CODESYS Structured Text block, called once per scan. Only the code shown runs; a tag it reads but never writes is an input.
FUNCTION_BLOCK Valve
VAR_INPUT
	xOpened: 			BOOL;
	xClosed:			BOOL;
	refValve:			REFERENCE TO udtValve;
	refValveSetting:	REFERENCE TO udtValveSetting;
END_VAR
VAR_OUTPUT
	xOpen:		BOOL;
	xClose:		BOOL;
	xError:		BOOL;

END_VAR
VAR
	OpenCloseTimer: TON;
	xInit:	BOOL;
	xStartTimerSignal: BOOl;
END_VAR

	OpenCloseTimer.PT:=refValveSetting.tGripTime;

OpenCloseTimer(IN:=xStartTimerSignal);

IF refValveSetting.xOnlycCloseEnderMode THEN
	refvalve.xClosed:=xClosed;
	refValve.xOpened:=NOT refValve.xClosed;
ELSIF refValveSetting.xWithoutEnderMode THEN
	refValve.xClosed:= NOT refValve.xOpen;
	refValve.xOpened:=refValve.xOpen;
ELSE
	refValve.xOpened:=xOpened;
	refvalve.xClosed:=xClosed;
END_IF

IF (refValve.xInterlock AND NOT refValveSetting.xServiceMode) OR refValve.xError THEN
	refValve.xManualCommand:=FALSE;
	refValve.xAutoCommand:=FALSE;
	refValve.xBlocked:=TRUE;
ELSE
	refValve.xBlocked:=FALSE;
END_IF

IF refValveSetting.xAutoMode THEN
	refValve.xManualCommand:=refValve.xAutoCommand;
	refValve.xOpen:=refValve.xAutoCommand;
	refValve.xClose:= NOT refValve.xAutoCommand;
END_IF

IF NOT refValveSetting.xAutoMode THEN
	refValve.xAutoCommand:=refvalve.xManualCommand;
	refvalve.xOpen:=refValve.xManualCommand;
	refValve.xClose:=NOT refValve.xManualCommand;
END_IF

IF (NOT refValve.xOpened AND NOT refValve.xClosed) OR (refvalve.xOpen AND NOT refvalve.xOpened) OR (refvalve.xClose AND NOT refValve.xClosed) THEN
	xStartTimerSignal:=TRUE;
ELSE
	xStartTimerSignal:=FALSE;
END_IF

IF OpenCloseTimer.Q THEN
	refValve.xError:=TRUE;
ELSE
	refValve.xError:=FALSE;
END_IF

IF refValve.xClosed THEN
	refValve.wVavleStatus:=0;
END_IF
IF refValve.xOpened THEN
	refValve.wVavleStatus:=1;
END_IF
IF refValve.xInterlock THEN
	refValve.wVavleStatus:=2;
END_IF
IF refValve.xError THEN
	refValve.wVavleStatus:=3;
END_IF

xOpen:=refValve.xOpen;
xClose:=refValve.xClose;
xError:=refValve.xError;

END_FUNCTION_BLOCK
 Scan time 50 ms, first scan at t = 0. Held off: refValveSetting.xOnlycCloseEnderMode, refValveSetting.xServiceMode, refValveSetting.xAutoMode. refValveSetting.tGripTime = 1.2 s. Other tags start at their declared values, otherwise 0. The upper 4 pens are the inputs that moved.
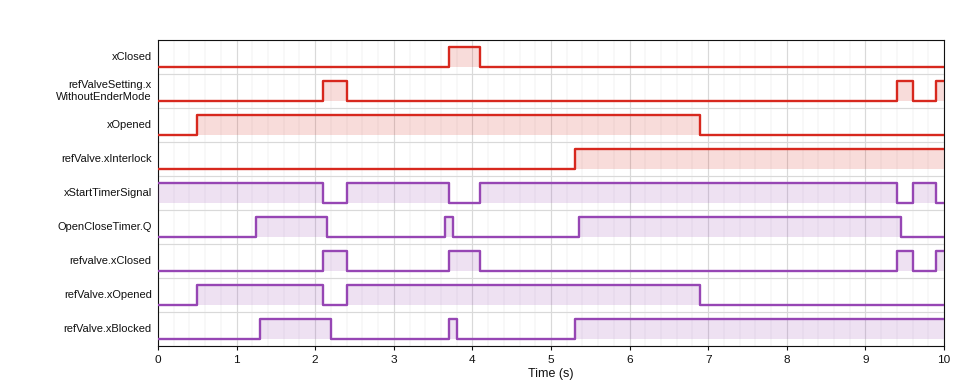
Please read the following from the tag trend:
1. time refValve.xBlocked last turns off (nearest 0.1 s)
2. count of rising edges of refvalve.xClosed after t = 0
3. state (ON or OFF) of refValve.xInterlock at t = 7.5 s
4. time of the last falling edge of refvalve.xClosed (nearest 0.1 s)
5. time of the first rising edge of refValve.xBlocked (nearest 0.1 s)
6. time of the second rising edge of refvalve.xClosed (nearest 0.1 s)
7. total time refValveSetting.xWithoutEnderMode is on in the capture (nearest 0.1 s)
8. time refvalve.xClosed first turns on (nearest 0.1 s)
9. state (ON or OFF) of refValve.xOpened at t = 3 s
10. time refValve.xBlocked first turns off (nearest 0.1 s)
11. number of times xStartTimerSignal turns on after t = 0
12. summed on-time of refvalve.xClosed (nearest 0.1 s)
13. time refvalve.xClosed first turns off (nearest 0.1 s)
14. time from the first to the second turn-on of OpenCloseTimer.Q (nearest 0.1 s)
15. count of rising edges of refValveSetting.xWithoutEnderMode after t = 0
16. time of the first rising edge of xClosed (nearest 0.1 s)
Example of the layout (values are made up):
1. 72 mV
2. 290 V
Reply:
1. 3.8 s
2. 4
3. ON
4. 9.6 s
5. 1.3 s
6. 3.7 s
7. 0.6 s
8. 2.1 s
9. ON
10. 2.2 s
11. 3
12. 1.0 s
13. 2.4 s
14. 2.4 s
15. 3
16. 3.7 s
